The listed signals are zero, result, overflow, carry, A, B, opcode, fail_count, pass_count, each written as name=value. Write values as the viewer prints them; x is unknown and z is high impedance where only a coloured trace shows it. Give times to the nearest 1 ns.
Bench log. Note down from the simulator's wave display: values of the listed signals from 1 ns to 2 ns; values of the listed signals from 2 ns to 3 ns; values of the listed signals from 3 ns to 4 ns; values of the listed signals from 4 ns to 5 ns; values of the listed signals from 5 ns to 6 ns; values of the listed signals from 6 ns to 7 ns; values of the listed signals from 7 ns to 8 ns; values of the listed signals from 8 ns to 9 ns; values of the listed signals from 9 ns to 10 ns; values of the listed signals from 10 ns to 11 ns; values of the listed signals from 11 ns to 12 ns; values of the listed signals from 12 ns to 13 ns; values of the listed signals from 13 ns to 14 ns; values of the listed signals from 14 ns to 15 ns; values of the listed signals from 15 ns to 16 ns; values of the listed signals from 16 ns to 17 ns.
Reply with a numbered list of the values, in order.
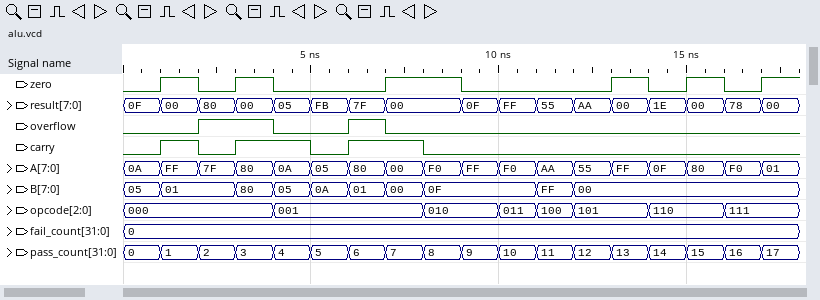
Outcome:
1. zero=1, result=00, overflow=0, carry=1, A=FF, B=01, opcode=000, fail_count=0, pass_count=1
2. zero=0, result=80, overflow=1, carry=0, A=7F, B=01, opcode=000, fail_count=0, pass_count=2
3. zero=1, result=00, overflow=1, carry=1, A=80, B=80, opcode=000, fail_count=0, pass_count=3
4. zero=0, result=05, overflow=0, carry=1, A=0A, B=05, opcode=001, fail_count=0, pass_count=4
5. zero=0, result=FB, overflow=0, carry=0, A=05, B=0A, opcode=001, fail_count=0, pass_count=5
6. zero=0, result=7F, overflow=1, carry=1, A=80, B=01, opcode=001, fail_count=0, pass_count=6
7. zero=1, result=00, overflow=0, carry=1, A=00, B=00, opcode=001, fail_count=0, pass_count=7
8. zero=1, result=00, overflow=0, carry=0, A=F0, B=0F, opcode=010, fail_count=0, pass_count=8
9. zero=0, result=0F, overflow=0, carry=0, A=FF, B=0F, opcode=010, fail_count=0, pass_count=9
10. zero=0, result=FF, overflow=0, carry=0, A=F0, B=0F, opcode=011, fail_count=0, pass_count=10
11. zero=0, result=55, overflow=0, carry=0, A=AA, B=FF, opcode=100, fail_count=0, pass_count=11
12. zero=0, result=AA, overflow=0, carry=0, A=55, B=00, opcode=101, fail_count=0, pass_count=12
13. zero=1, result=00, overflow=0, carry=0, A=FF, B=00, opcode=101, fail_count=0, pass_count=13
14. zero=0, result=1E, overflow=0, carry=0, A=0F, B=00, opcode=110, fail_count=0, pass_count=14
15. zero=1, result=00, overflow=0, carry=0, A=80, B=00, opcode=110, fail_count=0, pass_count=15
16. zero=0, result=78, overflow=0, carry=0, A=F0, B=00, opcode=111, fail_count=0, pass_count=16
